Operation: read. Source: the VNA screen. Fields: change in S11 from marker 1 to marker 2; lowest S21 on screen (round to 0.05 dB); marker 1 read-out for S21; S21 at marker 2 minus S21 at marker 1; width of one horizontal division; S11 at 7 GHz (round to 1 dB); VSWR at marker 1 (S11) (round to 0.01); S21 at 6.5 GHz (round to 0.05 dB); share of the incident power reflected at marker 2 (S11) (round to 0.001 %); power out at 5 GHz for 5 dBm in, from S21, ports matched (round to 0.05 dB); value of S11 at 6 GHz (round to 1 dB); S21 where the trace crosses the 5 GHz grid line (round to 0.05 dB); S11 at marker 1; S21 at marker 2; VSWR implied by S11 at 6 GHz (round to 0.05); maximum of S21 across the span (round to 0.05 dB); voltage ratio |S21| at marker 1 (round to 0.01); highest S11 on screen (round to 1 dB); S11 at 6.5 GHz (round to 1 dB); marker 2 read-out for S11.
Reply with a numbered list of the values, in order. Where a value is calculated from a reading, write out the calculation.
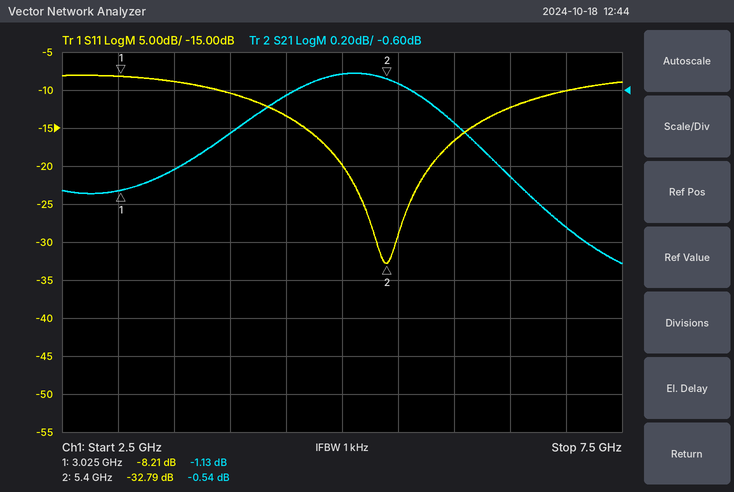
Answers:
1. -32.79 − (-8.21) = -24.58 dB
2. -1.50 dB
3. -1.13 dB
4. -0.54 − (-1.13) = 0.59 dB
5. 500 MHz
6. -10 dB
7. (1 + 0.3886)/(1 − 0.3886) ≈ 2.27
8. -1.05 dB
9. 10^(-32.79/10) ≈ 0.053 %
10. 5 dBm + (-0.50 dB) = 4.50 dBm
11. -17 dB
12. -0.50 dB
13. -8.21 dB
14. -0.54 dB
15. |Γ| = 10^(-17/20) = 0.1413; VSWR = (1 + 0.1413)/(1 − 0.1413) ≈ 1.33, so 1.35 to the nearest 0.05
16. -0.50 dB
17. 10^(-1.13/20) ≈ 0.88
18. -8 dB
19. -12 dB
20. -32.79 dB
